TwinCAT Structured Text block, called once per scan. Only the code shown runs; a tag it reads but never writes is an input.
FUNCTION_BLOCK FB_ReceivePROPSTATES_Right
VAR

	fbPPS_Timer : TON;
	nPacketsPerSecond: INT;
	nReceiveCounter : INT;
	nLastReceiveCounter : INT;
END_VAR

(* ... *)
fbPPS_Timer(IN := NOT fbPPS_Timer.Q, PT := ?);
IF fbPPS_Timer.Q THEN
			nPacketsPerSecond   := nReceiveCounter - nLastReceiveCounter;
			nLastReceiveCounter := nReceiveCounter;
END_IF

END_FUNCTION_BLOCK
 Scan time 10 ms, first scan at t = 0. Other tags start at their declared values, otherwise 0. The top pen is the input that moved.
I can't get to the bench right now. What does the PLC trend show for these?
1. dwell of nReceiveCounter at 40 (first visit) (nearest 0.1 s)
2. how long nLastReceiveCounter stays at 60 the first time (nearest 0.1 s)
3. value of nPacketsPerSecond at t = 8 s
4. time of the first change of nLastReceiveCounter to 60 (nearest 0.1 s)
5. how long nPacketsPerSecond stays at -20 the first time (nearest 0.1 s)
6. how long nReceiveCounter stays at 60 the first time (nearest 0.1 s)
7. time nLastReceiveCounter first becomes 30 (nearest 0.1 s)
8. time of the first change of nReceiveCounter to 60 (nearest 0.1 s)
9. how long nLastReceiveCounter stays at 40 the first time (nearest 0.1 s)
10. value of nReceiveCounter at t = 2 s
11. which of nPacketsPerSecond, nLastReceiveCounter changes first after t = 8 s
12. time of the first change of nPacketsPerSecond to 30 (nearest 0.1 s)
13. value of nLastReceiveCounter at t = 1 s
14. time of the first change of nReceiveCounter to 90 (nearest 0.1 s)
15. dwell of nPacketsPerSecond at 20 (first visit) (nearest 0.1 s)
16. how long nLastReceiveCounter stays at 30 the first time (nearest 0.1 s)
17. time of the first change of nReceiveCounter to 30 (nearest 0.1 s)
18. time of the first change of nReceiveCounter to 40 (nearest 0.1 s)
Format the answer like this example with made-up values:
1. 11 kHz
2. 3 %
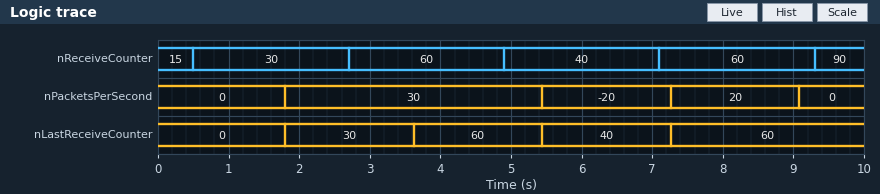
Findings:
1. 2.2 s
2. 1.8 s
3. 20
4. 3.6 s
5. 1.8 s
6. 2.2 s
7. 1.8 s
8. 2.7 s
9. 1.8 s
10. 30
11. nPacketsPerSecond
12. 1.8 s
13. 0
14. 9.3 s
15. 1.8 s
16. 1.8 s
17. 0.5 s
18. 4.9 s
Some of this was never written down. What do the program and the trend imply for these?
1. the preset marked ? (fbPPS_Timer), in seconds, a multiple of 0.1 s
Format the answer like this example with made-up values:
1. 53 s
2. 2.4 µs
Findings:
1. 1.8 s
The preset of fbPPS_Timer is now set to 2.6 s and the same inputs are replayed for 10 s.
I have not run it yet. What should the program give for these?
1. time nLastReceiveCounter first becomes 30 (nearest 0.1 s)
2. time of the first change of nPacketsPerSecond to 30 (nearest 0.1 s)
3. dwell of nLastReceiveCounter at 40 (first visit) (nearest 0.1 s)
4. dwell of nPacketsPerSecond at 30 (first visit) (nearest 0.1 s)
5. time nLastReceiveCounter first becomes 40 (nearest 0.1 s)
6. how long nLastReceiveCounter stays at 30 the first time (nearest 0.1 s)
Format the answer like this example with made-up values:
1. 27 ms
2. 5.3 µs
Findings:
1. 2.6 s
2. 2.6 s
3. 2.6 s
4. 2.6 s
5. 5.2 s
6. 2.6 s
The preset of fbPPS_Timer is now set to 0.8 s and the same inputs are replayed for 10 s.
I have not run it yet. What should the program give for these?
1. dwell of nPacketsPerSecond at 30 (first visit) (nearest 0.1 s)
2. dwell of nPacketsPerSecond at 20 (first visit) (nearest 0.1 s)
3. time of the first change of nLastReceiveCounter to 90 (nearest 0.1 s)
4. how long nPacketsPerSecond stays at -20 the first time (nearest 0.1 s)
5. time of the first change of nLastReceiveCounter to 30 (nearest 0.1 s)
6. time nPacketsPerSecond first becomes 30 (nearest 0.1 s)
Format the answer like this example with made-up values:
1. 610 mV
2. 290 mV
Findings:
1. 0.8 s
2. 0.8 s
3. 9.8 s
4. 0.8 s
5. 0.8 s
6. 0.8 s
